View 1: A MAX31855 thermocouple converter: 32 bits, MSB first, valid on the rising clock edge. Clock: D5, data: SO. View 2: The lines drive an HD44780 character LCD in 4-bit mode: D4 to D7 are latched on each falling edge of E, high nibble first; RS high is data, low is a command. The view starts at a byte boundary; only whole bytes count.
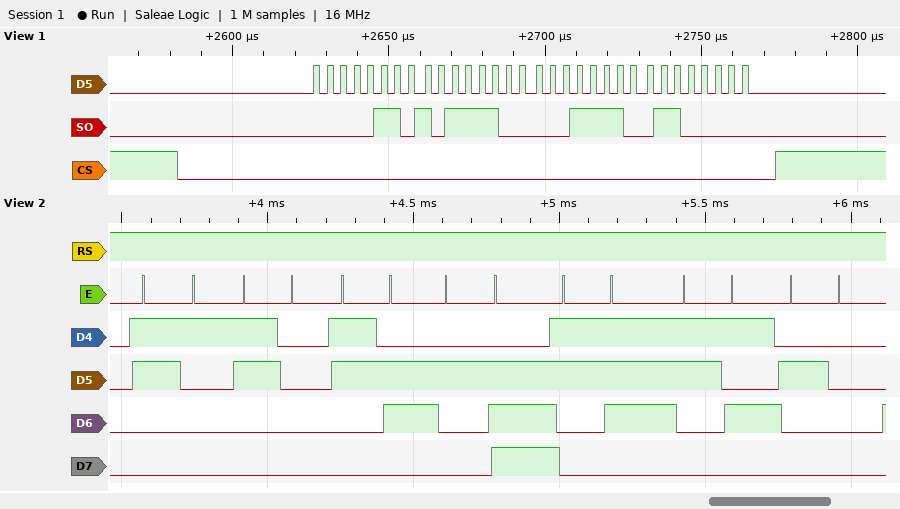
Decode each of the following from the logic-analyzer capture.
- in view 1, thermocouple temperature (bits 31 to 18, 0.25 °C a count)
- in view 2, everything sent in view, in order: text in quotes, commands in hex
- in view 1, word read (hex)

107.75 °C
"106.75 "
0x06BC1E60
